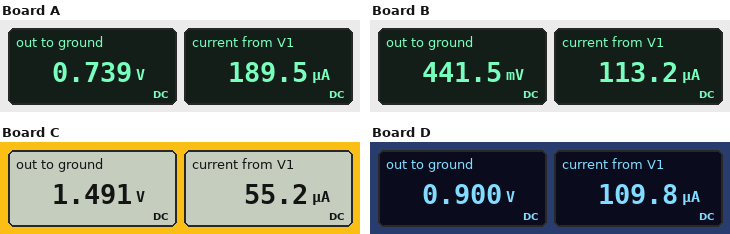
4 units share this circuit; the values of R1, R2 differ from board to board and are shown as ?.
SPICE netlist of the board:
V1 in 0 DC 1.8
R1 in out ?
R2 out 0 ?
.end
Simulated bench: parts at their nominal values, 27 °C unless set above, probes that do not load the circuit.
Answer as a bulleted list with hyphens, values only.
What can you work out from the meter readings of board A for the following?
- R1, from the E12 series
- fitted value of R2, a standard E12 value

- 5.6 kΩ
- 3.9 kΩ
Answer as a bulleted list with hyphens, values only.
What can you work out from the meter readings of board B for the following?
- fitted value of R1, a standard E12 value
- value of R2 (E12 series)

- 12 kΩ
- 3.9 kΩ
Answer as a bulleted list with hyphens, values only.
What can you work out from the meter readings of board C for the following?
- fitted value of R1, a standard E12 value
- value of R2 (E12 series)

- 5.6 kΩ
- 27 kΩ
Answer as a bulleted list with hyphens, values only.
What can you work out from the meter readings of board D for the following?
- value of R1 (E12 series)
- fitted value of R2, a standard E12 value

- 8.2 kΩ
- 8.2 kΩ
